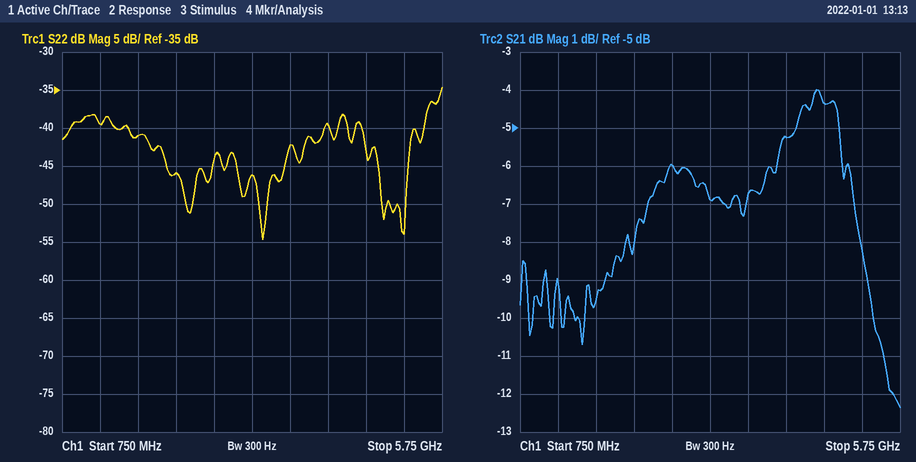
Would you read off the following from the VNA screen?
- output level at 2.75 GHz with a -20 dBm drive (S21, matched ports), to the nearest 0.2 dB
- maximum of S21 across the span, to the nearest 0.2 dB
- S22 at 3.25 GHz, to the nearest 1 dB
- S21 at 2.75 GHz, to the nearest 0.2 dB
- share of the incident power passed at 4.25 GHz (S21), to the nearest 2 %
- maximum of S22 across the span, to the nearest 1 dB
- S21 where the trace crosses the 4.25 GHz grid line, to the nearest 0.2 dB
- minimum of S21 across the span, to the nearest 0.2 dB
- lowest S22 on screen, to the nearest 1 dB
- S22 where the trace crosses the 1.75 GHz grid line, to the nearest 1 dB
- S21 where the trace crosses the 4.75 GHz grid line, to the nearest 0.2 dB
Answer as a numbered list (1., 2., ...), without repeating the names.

1. -26.0 dBm
2. -4.0 dB
3. -46 dB
4. -6.0 dB
5. 30 %
6. -35 dB
7. -5.2 dB
8. -12.4 dB
9. -55 dB
10. -41 dB
11. -4.4 dB
